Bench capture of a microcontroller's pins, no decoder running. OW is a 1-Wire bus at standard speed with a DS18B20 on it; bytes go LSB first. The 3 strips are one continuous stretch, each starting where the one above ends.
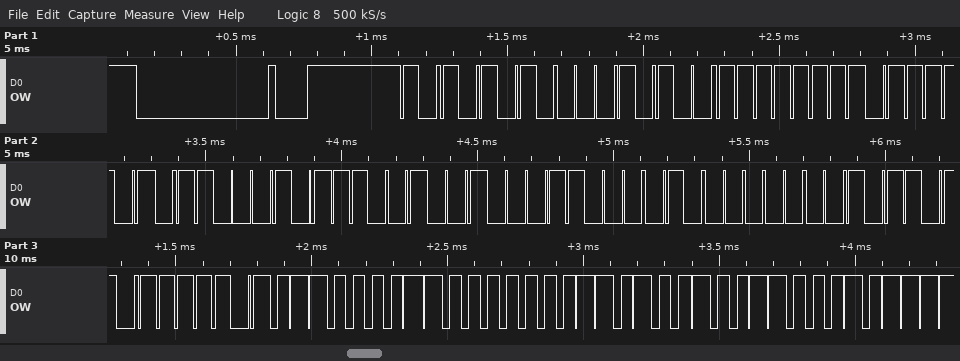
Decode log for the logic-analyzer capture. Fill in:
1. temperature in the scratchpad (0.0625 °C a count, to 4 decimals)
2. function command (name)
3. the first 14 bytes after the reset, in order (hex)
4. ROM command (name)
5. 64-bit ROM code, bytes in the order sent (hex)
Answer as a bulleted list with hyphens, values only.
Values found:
- 24.3750 °C
- Read Scratchpad
- 55 28 FF 5E A3 93 18 02 B4 BE 86 01 4B 46
- Match ROM
- 28 FF 5E A3 93 18 02 B4
